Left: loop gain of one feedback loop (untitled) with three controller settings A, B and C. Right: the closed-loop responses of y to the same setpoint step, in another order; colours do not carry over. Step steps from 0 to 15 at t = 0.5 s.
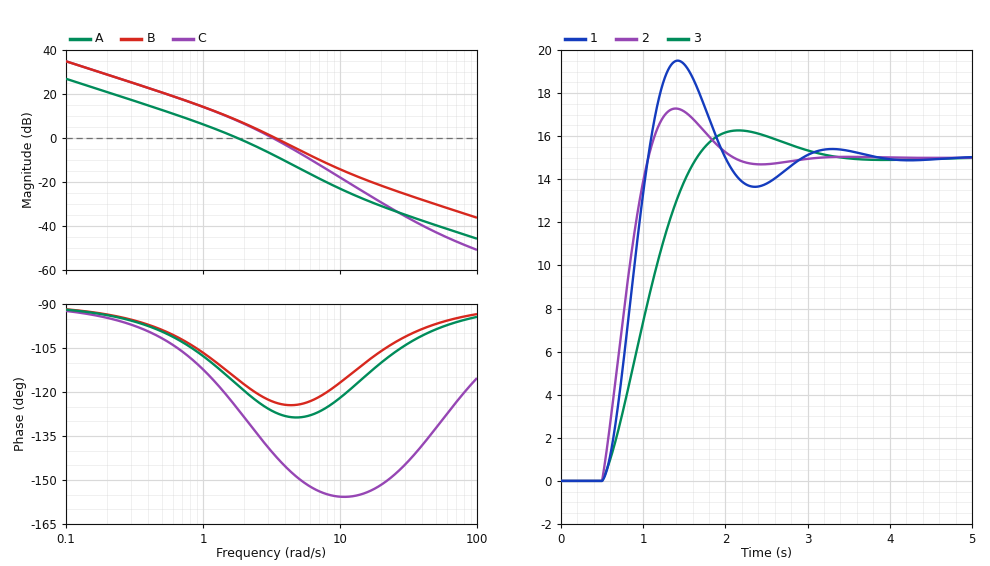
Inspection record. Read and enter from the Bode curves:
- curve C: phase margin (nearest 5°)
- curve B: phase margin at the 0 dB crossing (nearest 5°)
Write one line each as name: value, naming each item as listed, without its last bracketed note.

curve C: phase margin: 40°
curve B: phase margin at the 0 dB crossing: 55°
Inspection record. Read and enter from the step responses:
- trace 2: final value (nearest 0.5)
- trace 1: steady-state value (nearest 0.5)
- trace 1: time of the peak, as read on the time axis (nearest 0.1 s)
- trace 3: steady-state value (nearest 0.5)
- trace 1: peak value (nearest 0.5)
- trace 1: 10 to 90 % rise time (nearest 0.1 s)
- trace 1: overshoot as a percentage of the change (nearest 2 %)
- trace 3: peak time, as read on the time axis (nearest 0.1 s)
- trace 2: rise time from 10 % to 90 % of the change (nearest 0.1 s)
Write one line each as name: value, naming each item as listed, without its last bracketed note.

trace 2: final value: 15.0
trace 1: steady-state value: 15.0
trace 1: time of the peak, as read on the time axis: 1.4 s
trace 3: steady-state value: 15.0
trace 1: peak value: 19.5
trace 1: 10 to 90 % rise time: 0.4 s
trace 1: overshoot as a percentage of the change: 30 %
trace 3: peak time, as read on the time axis: 2.2 s
trace 2: rise time from 10 % to 90 % of the change: 0.4 s
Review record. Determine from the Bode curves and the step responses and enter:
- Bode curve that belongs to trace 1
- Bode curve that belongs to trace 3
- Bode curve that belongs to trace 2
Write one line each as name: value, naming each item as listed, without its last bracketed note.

Bode curve that belongs to trace 1: C
Bode curve that belongs to trace 3: A
Bode curve that belongs to trace 2: B
